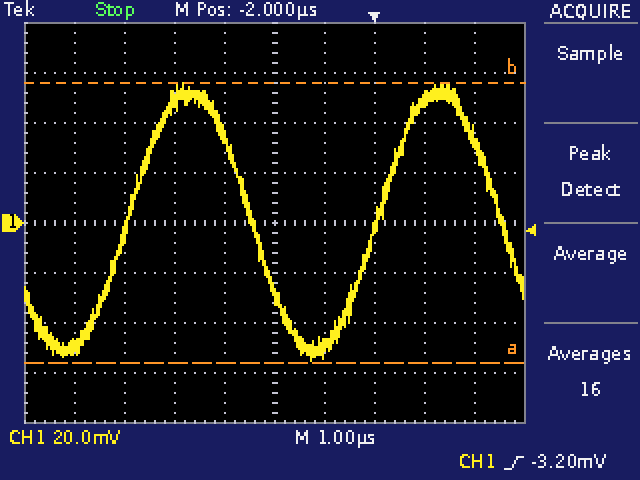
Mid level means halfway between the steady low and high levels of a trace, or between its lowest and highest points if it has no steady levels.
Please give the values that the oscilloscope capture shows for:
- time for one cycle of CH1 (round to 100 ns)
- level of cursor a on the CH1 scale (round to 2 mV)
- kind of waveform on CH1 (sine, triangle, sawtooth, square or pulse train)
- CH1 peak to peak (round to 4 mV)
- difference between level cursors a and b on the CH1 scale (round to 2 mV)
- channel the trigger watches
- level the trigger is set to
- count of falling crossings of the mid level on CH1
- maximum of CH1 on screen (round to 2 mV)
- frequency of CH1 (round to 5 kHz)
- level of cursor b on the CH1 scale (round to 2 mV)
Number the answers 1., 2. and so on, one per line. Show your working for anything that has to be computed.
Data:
1. 5.0 µs
2. -56 mV
3. sine
4. 112 mV
5. 112 mV
6. CH1
7. -3.20 mV
8. 2
9. 56 mV
10. 1 / 5.0 µs ≈ 200 kHz
11. 56 mV
